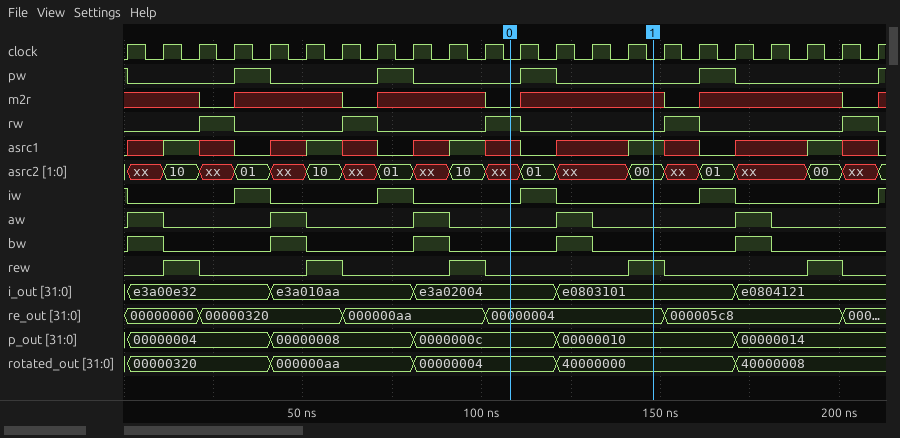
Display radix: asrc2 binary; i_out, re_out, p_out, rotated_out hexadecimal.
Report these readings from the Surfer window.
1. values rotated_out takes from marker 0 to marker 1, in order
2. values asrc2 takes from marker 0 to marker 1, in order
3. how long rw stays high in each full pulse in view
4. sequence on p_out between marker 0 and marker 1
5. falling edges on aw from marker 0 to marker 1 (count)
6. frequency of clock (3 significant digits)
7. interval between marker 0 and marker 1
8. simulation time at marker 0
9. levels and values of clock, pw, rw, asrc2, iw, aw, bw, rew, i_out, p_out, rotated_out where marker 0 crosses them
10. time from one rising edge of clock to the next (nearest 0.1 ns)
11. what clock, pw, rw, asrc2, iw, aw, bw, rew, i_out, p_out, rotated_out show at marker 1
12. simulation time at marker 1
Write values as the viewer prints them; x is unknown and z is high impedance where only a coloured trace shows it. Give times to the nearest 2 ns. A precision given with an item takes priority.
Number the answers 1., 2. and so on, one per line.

1. 00000004, 40000000
2. xx, 01, xx, 00
3. 10 ns, 10 ns, 10 ns, 10 ns, 10 ns
4. 0000000c, 00000010
5. 1
6. 100 MHz
7. 40 ns
8. 108 ns
9. clock=0, pw=0, rw=1, asrc2=xx, iw=0, aw=0, bw=0, rew=0, i_out=e3a02004, p_out=0000000c, rotated_out=00000004
10. 10 ns
11. clock=0, pw=0, rw=0, asrc2=00, iw=0, aw=0, bw=0, rew=1, i_out=e0803101, p_out=00000010, rotated_out=40000000
12. 148 ns
